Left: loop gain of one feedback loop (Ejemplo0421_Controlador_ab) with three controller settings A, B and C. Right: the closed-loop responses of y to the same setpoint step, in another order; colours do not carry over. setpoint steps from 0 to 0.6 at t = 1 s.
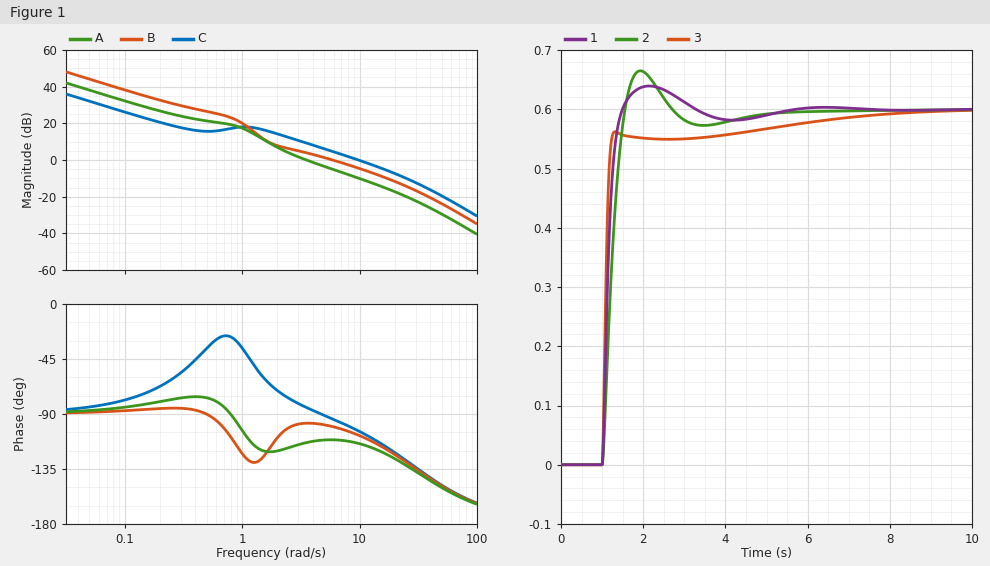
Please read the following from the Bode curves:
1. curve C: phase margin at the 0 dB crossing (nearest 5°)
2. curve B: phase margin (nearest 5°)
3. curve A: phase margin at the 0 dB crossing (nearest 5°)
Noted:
75°
80°
65°
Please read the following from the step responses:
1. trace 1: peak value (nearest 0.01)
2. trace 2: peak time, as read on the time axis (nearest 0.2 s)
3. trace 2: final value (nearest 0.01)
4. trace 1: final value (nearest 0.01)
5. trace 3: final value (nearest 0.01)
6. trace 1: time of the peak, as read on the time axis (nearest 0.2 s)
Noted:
0.64
2.0 s
0.60
0.60
0.60
2.2 s
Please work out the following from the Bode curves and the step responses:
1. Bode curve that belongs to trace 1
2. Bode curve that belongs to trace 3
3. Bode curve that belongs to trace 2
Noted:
B
C
A
